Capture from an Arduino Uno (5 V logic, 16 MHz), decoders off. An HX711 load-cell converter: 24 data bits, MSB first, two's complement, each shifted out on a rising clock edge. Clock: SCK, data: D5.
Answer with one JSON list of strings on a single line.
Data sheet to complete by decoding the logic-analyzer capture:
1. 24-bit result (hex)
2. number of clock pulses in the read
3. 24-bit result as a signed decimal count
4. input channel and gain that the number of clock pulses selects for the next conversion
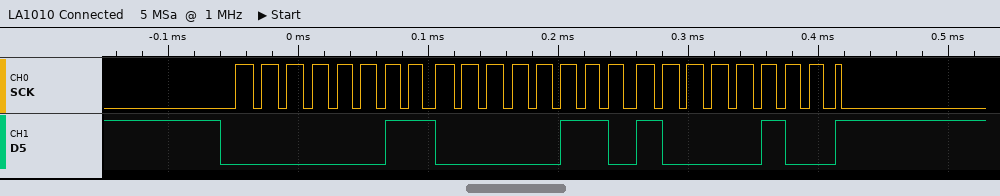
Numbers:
["0x030684", "25", "198276", "channel A, gain 128"]
